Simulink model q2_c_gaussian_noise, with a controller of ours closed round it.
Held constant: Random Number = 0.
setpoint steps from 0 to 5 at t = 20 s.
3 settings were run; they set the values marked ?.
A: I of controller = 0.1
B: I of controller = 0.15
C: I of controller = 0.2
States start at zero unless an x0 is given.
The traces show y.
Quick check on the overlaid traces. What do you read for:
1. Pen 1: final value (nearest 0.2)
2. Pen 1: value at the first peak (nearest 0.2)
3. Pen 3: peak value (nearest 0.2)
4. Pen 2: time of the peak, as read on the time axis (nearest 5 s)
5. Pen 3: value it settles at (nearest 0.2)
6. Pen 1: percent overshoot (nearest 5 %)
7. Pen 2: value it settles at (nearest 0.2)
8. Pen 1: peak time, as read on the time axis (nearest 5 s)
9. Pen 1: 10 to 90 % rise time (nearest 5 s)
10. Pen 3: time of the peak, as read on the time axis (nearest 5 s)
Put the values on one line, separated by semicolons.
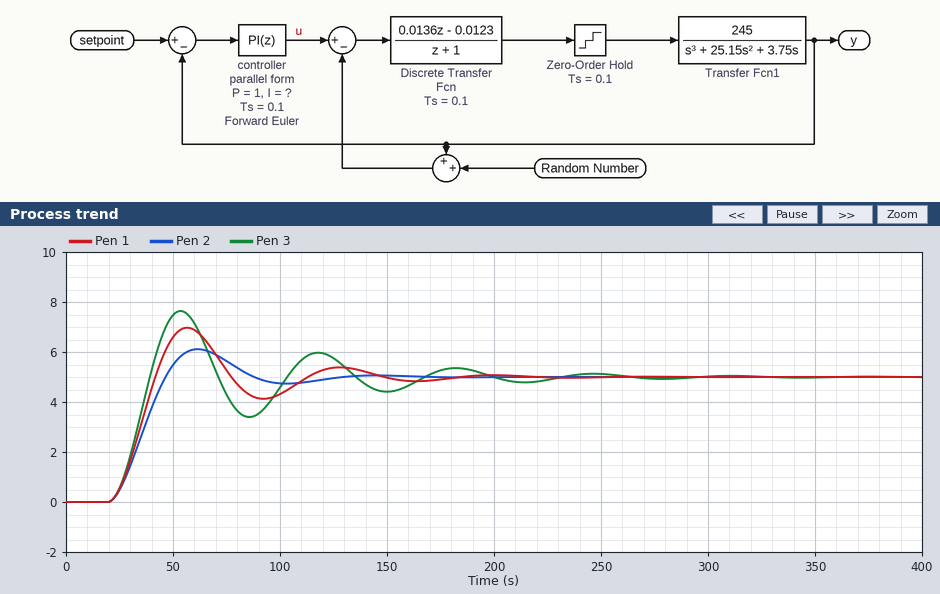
5.0; 7.0; 7.6; 60 s; 5.0; 40 %; 5.0; 55 s; 15 s; 55 s
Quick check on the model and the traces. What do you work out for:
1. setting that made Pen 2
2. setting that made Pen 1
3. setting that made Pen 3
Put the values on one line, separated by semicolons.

A; B; C
